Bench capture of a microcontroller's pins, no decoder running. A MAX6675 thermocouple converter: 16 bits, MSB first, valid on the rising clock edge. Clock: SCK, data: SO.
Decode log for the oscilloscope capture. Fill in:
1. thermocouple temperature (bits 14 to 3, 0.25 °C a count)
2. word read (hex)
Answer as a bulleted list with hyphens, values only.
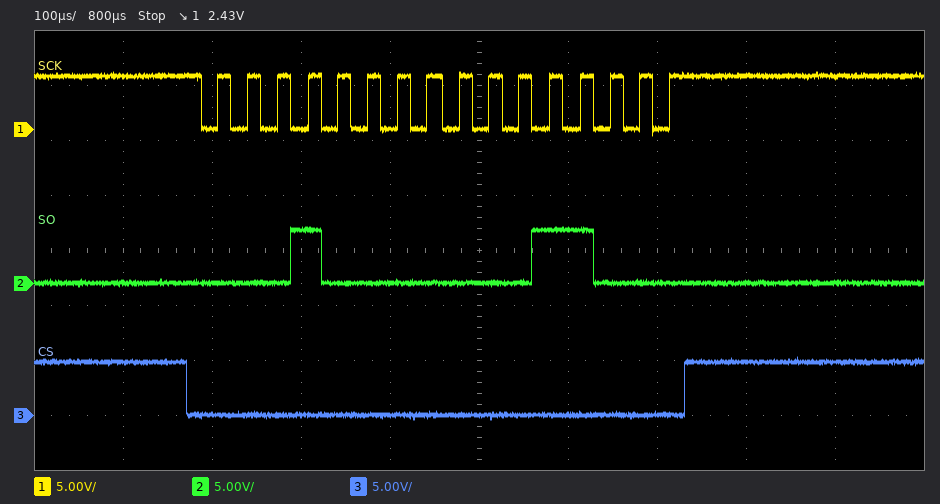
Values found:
- 128.75 °C
- 0x1018
